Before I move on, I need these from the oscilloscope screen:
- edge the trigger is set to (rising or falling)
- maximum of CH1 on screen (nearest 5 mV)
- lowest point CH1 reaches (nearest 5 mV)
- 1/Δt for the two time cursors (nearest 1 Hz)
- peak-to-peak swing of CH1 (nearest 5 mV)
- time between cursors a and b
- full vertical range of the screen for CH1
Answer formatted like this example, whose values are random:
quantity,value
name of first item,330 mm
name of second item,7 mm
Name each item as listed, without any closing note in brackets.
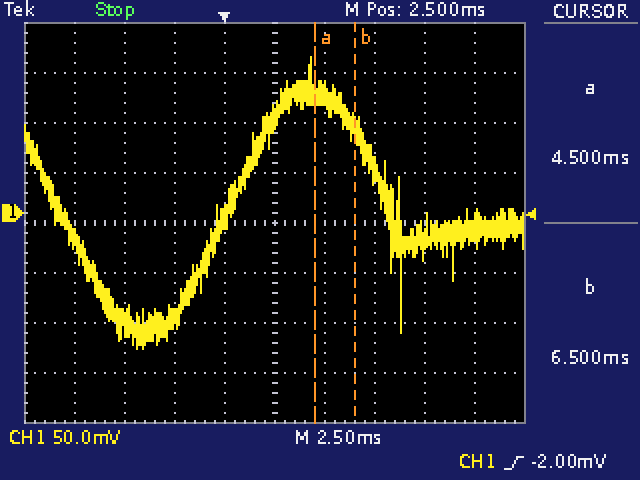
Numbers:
quantity,value
edge the trigger is set to,rising
maximum of CH1 on screen,155 mV
lowest point CH1 reaches,-135 mV
1/Δt for the two time cursors,500 Hz
peak-to-peak swing of CH1,290 mV
time between cursors a and b,2.00 ms
full vertical range of the screen for CH1,400 mV
